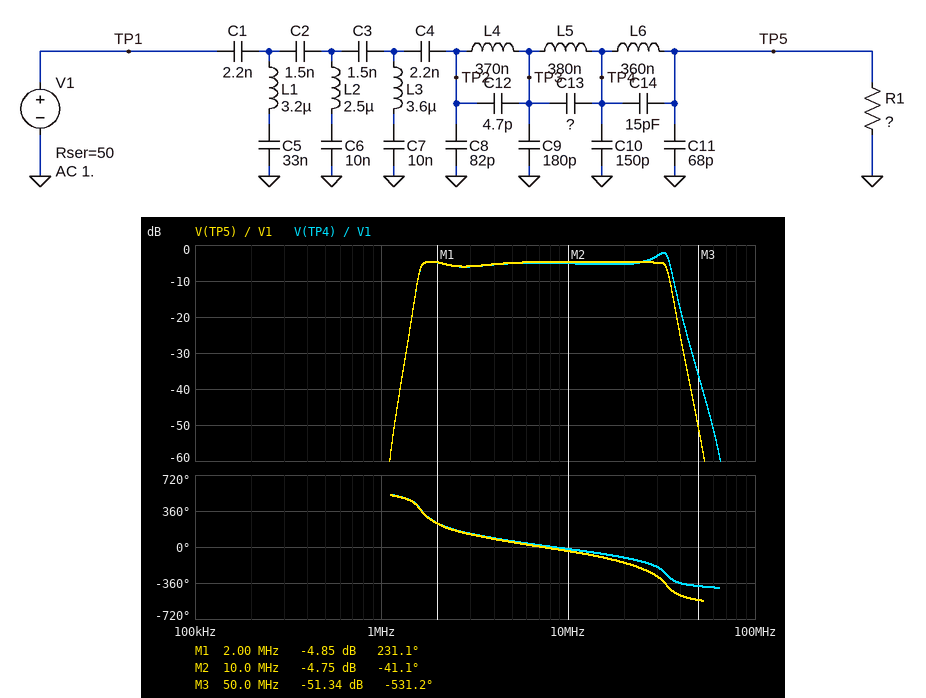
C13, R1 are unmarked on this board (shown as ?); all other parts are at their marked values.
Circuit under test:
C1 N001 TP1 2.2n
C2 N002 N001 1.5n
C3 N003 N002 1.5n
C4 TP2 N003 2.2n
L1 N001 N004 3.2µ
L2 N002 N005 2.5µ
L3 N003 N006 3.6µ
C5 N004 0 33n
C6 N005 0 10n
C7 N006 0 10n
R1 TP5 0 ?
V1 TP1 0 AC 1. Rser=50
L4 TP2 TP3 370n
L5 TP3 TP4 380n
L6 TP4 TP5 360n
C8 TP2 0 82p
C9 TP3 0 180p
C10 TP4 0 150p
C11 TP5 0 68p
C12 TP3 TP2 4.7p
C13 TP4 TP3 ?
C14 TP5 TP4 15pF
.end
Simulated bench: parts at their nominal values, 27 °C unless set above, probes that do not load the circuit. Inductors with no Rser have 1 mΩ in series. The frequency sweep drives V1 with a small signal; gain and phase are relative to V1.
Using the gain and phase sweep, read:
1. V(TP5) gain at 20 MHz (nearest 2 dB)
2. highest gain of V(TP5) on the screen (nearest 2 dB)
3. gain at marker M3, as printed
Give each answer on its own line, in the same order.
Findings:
-4 dB
-4 dB
-51.34 dB
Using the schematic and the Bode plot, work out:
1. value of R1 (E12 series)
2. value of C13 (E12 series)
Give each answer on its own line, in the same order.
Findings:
68 Ω
12 pF
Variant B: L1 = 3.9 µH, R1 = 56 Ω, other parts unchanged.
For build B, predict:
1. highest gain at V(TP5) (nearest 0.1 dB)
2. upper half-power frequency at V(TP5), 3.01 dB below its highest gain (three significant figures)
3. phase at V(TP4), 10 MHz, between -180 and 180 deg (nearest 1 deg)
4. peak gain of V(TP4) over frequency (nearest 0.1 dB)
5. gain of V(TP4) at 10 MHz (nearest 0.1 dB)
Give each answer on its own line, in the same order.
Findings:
-5.5 dB
34.0 MHz
-18 deg
-1.2 dB
-5.6 dB
